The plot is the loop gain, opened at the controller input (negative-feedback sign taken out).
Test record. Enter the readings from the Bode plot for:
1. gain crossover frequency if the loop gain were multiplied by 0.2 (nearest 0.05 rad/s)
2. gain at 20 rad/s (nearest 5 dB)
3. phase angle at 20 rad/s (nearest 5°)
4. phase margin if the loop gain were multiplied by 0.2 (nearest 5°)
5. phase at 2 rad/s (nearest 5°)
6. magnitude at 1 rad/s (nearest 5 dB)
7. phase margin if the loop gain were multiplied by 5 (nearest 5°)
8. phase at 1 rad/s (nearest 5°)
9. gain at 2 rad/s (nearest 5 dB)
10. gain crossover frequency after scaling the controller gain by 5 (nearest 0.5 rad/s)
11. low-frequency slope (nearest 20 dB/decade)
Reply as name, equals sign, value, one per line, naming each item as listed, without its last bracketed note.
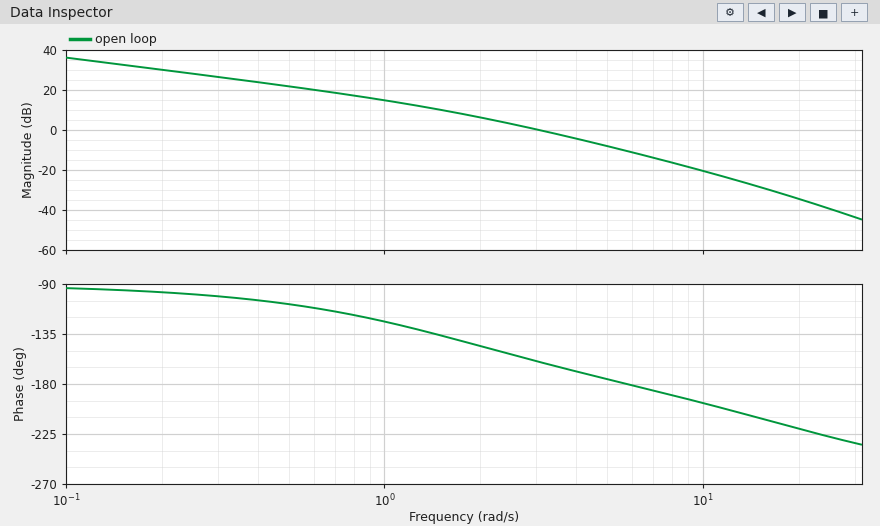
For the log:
gain crossover frequency if the loop gain were multiplied by 0.2 = 1.10 rad/s
gain at 20 rad/s = -35 dB
phase angle at 20 rad/s = -220°
phase margin if the loop gain were multiplied by 0.2 = 55°
phase at 2 rad/s = -145°
magnitude at 1 rad/s = 15 dB
phase margin if the loop gain were multiplied by 5 = -5°
phase at 1 rad/s = -125°
gain at 2 rad/s = 5 dB
gain crossover frequency after scaling the controller gain by 5 = 7.0 rad/s
low-frequency slope = -20 dB/decade
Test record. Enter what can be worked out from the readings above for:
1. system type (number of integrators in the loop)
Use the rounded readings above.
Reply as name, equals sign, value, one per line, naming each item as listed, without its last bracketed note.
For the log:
system type = 1
